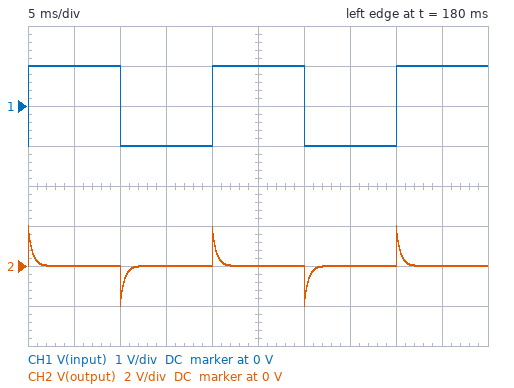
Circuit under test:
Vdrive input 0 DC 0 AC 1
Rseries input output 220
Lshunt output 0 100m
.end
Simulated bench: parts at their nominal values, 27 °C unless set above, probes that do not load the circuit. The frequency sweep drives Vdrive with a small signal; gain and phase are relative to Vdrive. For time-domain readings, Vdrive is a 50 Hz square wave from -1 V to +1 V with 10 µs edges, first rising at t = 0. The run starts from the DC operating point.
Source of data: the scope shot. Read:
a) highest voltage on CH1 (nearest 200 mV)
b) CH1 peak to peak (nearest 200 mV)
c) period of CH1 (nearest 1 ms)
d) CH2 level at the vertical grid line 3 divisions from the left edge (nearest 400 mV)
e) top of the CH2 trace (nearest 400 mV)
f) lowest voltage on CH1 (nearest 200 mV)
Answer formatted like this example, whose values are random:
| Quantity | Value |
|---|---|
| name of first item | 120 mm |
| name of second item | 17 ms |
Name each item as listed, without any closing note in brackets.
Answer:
| Quantity | Value |
|---|---|
| highest voltage on CH1 | 1.0 V |
| CH1 peak to peak | 2.0 V |
| period of CH1 | 20 ms |
| CH2 level at the vertical grid line 3 divisions from the left edge | 0 V |
| top of the CH2 trace | 2.0 V |
| lowest voltage on CH1 | -1.0 V |
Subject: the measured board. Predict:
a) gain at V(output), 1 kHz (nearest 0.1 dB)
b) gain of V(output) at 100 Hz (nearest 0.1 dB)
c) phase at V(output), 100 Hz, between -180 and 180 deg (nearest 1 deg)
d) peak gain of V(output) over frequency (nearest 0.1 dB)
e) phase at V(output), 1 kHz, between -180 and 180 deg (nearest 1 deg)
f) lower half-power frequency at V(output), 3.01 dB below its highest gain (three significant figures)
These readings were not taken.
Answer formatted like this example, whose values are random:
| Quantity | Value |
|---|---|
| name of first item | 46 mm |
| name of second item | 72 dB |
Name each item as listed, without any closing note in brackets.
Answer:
| Quantity | Value |
|---|---|
| gain at V(output), 1 kHz | -0.5 dB |
| gain of V(output) at 100 Hz | -11.2 dB |
| phase at V(output), 100 Hz, between -180 and 180 deg | 74 deg |
| peak gain of V(output) over frequency | 0 dB |
| phase at V(output), 1 kHz, between -180 and 180 deg | 19 deg |
| lower half-power frequency at V(output), 3.01 dB below its highest gain | 350 Hz |
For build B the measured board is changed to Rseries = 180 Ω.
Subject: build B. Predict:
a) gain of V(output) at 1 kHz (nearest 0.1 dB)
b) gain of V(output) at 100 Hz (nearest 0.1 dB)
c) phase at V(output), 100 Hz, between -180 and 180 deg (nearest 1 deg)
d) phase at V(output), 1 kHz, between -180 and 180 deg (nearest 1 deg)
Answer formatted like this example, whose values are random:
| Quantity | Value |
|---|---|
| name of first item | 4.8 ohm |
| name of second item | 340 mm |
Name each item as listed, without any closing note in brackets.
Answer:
| Quantity | Value |
|---|---|
| gain of V(output) at 1 kHz | -0.3 dB |
| gain of V(output) at 100 Hz | -9.6 dB |
| phase at V(output), 100 Hz, between -180 and 180 deg | 71 deg |
| phase at V(output), 1 kHz, between -180 and 180 deg | 16 deg |
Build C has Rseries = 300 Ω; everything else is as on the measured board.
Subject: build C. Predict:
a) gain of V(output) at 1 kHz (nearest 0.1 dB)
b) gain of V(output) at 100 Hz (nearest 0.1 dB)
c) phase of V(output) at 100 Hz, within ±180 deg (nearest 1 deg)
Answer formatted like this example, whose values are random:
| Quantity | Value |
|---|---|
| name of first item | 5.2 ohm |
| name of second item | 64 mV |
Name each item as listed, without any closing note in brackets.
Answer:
| Quantity | Value |
|---|---|
| gain of V(output) at 1 kHz | -0.9 dB |
| gain of V(output) at 100 Hz | -13.8 dB |
| phase of V(output) at 100 Hz, within ±180 deg | 78 deg |
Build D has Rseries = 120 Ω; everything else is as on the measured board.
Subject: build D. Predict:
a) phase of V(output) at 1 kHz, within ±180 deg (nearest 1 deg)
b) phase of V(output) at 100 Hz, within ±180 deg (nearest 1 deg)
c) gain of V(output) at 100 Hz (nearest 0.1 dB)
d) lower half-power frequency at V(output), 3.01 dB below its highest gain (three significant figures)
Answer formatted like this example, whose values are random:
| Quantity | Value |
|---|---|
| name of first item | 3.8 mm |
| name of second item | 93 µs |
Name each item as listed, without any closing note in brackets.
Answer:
| Quantity | Value |
|---|---|
| phase of V(output) at 1 kHz, within ±180 deg | 11 deg |
| phase of V(output) at 100 Hz, within ±180 deg | 62 deg |
| gain of V(output) at 100 Hz | -6.7 dB |
| lower half-power frequency at V(output), 3.01 dB below its highest gain | 191 Hz |
